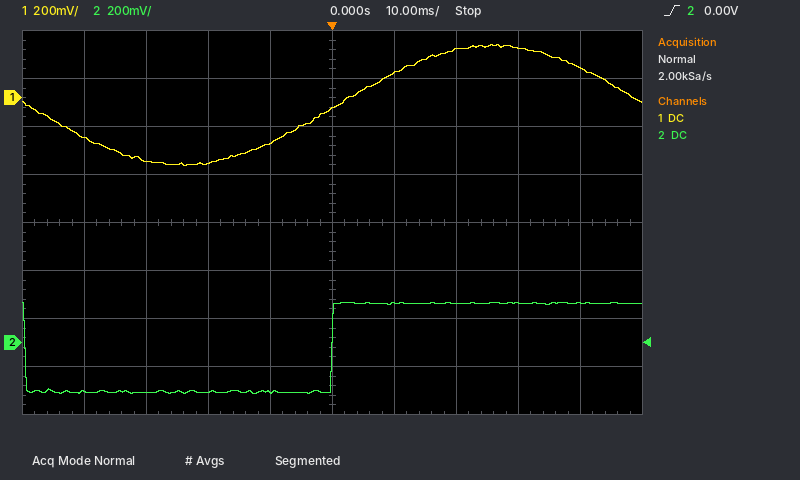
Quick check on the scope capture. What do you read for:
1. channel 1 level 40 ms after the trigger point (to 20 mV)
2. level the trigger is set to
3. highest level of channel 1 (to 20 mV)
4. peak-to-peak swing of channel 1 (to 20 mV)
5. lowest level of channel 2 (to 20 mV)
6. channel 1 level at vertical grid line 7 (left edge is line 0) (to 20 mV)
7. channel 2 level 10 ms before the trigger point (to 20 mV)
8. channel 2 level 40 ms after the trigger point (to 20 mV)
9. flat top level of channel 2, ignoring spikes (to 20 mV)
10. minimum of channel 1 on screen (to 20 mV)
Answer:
120 mV
0.00 V
220 mV
500 mV
-220 mV
200 mV
-200 mV
160 mV
160 mV
-280 mV
